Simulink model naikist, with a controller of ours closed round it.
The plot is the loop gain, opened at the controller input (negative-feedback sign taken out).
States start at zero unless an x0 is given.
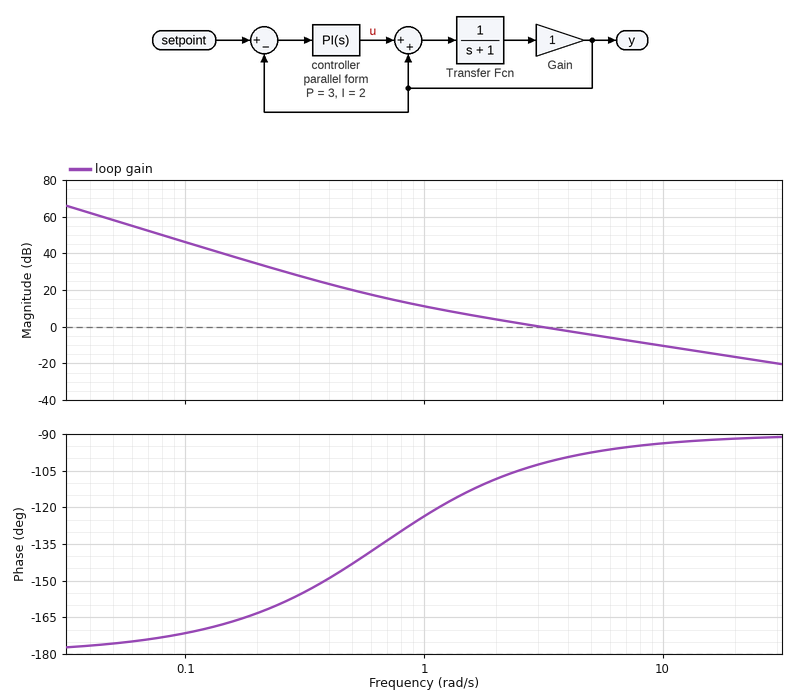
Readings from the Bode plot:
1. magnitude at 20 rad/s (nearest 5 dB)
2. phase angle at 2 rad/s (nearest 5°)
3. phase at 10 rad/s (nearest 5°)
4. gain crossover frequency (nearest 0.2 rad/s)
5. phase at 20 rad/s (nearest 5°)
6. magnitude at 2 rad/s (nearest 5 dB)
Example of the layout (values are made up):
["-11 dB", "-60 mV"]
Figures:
["-15 dB", "-110°", "-95°", "3.0 rad/s", "-90°", "5 dB"]
